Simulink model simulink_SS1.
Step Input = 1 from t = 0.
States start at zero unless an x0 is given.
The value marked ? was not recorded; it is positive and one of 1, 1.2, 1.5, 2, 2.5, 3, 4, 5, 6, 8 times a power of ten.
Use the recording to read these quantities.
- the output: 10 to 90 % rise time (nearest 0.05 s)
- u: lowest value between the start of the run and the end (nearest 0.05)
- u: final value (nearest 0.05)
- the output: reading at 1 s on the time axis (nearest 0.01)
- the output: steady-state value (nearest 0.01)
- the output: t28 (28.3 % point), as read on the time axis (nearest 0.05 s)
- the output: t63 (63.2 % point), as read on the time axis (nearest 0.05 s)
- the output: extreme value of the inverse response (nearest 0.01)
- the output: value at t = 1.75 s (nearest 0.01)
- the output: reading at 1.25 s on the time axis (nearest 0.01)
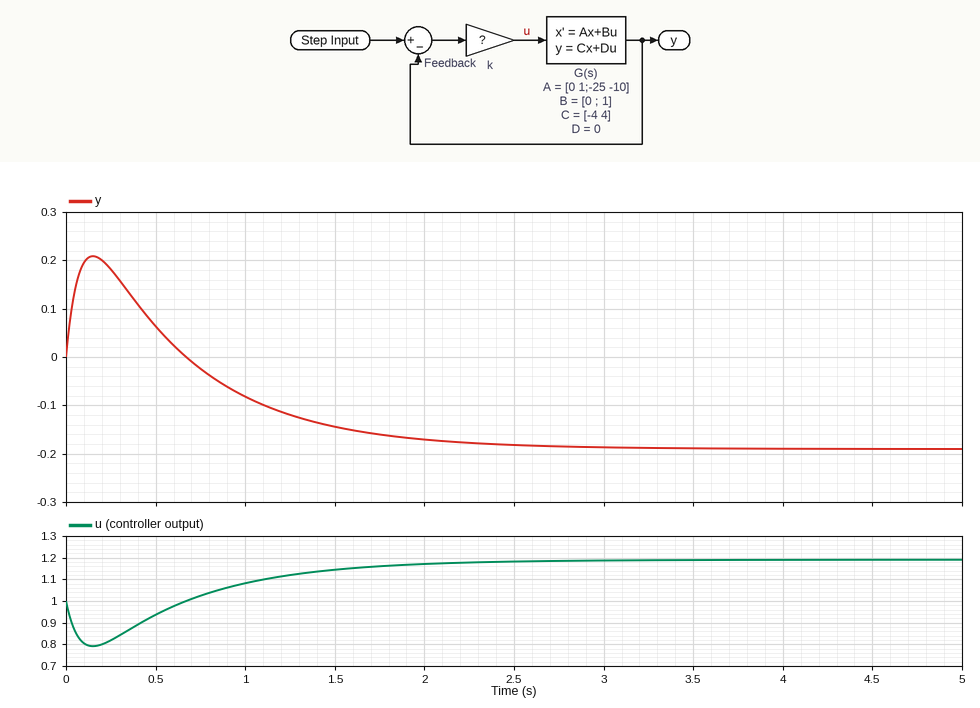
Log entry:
1.30 s
0.80
1.20
-0.08
-0.19
0.85 s
1.25 s
0.21
-0.16
-0.12
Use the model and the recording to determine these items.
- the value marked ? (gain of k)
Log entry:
1
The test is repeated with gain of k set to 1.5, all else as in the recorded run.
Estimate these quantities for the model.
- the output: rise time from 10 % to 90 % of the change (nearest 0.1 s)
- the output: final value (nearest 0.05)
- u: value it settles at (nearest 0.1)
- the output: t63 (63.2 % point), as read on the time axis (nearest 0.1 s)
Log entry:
1.7 s
-0.30
2.0
1.5 s
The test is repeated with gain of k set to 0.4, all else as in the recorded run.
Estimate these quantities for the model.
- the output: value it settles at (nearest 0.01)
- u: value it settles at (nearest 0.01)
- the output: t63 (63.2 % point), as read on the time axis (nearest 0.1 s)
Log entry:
-0.07
0.43
1.0 s
